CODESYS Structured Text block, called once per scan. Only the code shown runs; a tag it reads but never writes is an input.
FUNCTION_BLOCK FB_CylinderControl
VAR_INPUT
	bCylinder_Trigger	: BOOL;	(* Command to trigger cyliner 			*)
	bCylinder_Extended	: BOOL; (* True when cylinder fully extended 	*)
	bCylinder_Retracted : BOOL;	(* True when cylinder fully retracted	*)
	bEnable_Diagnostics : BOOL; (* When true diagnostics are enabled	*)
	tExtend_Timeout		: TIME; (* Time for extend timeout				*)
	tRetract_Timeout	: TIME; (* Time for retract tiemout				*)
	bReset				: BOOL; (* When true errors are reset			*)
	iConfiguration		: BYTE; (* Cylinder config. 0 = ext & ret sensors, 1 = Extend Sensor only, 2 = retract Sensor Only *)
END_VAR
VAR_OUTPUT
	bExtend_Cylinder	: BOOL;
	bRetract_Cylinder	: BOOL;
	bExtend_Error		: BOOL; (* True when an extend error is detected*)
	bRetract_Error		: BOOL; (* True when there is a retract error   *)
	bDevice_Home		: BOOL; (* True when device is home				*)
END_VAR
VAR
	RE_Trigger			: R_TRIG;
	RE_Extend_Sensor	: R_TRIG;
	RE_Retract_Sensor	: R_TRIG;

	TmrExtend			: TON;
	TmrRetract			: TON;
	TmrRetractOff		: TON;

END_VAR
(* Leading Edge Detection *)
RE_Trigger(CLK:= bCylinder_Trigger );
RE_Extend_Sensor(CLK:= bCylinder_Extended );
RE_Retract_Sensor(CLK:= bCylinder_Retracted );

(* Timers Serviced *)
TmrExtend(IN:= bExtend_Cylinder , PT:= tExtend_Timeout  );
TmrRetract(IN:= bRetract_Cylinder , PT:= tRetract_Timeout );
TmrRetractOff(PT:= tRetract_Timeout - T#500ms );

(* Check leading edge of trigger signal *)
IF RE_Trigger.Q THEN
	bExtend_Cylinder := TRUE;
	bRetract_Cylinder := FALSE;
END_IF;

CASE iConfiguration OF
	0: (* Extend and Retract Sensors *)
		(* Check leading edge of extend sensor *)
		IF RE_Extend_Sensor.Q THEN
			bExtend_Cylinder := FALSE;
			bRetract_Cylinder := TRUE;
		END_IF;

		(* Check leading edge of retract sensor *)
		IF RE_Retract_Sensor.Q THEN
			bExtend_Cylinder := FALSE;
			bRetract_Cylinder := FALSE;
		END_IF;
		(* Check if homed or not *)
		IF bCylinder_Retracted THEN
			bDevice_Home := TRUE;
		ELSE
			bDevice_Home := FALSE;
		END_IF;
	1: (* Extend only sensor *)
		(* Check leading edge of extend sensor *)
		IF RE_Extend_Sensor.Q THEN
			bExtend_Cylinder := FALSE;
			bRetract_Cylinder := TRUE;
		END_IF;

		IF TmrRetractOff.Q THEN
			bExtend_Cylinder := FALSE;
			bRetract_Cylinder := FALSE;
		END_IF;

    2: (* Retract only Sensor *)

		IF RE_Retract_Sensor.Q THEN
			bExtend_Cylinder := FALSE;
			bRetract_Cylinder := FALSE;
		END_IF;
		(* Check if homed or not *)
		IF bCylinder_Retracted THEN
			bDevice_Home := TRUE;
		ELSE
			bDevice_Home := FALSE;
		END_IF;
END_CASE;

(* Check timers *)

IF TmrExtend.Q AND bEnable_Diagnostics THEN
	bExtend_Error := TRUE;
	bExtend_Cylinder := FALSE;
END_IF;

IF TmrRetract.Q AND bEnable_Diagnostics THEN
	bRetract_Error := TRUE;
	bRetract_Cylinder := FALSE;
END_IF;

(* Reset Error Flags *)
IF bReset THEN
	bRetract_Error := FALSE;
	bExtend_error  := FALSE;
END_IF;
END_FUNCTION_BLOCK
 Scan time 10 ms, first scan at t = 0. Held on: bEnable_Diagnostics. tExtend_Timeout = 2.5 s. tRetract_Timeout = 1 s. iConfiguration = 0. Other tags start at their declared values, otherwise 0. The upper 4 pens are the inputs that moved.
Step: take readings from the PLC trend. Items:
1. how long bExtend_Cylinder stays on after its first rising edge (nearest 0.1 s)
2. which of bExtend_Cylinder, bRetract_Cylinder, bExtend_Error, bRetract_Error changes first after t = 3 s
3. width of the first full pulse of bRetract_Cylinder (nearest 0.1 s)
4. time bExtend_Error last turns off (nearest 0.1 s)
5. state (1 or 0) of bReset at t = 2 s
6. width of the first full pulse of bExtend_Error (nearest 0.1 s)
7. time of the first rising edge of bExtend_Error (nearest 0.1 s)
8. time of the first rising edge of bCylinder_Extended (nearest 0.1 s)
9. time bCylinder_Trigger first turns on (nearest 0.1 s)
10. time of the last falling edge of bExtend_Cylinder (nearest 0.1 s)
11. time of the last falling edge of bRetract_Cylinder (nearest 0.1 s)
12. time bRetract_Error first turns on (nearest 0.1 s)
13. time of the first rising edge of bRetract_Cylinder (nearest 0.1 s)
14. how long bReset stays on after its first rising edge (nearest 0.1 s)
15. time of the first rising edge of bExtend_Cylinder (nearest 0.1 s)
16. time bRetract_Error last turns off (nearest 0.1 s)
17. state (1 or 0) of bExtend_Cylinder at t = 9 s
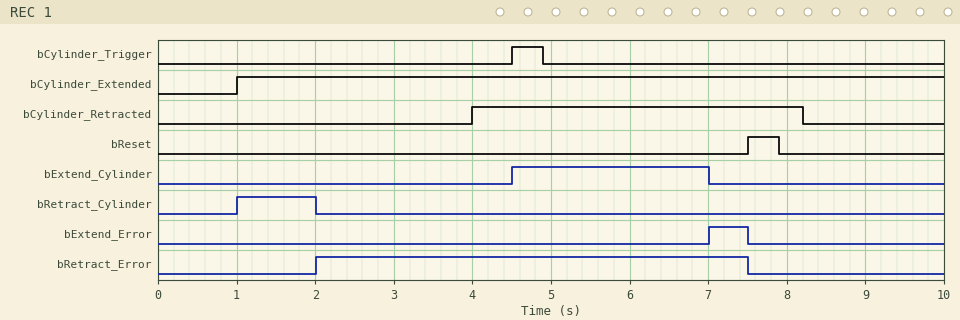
2.5 s
bExtend_Cylinder
1.0 s
7.5 s
0
0.5 s
7.0 s
1.0 s
4.5 s
7.0 s
2.0 s
2.0 s
1.0 s
0.4 s
4.5 s
7.5 s
0
